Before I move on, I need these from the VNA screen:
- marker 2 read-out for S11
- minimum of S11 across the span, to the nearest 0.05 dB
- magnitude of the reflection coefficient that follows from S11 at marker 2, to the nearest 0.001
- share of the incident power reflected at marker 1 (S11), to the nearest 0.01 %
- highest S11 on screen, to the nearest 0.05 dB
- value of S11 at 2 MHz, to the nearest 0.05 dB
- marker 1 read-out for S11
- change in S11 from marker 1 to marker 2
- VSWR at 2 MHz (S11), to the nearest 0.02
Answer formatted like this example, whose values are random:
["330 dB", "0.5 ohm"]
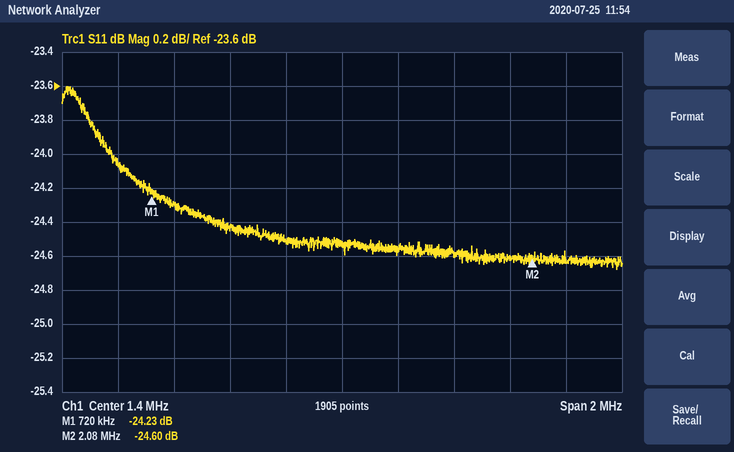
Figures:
["-24.60 dB", "-24.70 dB", "0.059", "0.38 %", "-23.60 dB", "-24.60 dB", "-24.23 dB", "-0.37 dB", "1.12"]
